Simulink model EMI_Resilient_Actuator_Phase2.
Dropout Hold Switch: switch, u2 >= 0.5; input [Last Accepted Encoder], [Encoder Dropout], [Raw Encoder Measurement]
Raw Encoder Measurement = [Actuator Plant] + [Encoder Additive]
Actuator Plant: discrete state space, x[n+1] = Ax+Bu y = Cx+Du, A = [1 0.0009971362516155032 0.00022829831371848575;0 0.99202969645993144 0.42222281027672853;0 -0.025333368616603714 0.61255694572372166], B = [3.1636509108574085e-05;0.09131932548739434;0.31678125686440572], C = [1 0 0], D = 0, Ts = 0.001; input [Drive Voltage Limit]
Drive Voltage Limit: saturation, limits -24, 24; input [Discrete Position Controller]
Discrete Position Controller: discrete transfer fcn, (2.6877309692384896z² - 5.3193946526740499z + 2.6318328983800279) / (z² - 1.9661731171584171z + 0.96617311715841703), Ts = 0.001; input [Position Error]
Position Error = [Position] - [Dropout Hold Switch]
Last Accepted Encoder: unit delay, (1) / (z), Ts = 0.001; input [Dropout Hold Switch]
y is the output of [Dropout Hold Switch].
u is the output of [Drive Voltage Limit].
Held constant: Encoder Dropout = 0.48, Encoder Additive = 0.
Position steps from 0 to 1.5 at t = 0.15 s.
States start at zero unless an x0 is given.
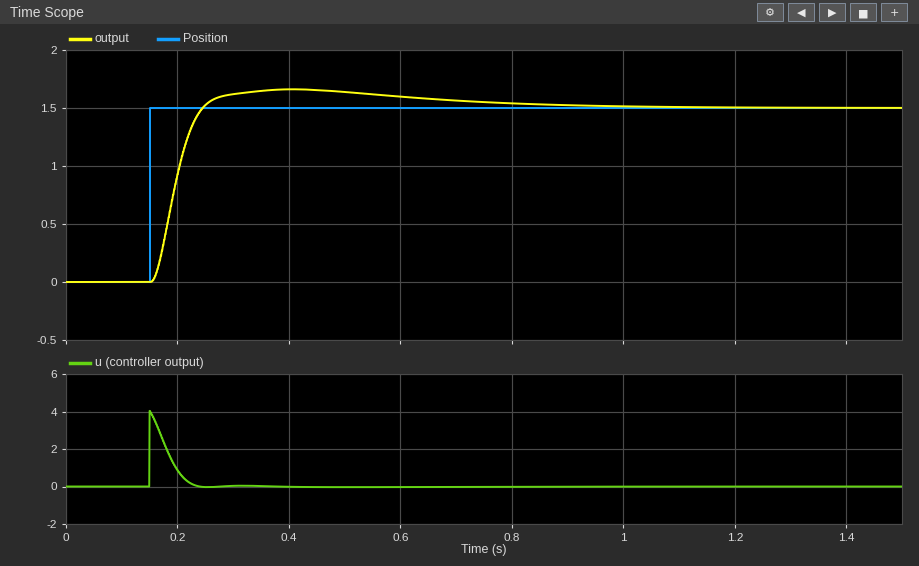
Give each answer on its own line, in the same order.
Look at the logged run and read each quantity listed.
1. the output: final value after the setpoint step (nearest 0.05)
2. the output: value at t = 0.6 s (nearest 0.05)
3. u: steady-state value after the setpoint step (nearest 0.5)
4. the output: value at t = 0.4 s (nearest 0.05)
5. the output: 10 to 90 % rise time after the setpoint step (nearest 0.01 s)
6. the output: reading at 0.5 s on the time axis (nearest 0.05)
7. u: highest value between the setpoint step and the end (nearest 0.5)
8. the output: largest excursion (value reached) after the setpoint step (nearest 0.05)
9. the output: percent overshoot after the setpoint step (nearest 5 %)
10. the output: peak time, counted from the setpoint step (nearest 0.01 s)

1.50
1.60
0.0
1.65
0.06 s
1.65
4.0
1.65
10 %
0.26 s
